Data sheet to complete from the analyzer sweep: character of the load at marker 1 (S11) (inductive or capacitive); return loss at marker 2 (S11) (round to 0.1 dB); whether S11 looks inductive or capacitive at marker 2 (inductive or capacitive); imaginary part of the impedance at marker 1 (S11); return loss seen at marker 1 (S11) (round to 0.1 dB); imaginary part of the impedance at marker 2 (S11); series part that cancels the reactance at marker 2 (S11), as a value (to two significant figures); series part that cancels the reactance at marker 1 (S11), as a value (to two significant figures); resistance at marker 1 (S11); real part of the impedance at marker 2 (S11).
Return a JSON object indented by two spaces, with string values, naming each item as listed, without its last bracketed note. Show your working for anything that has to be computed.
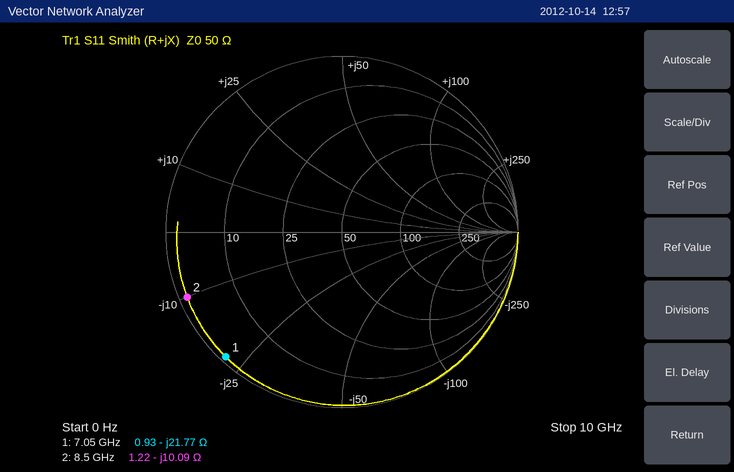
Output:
{
  "character of the load at marker 1 (S11)": "capacitive",
  "return loss at marker 2 (S11)": "0.4 dB",
  "whether S11 looks inductive or capacitive at marker 2": "capacitive",
  "imaginary part of the impedance at marker 1": "-21.77 Ω",
  "return loss seen at marker 1 (S11)": "0.3 dB",
  "imaginary part of the impedance at marker 2": "-10.09 Ω",
  "series part that cancels the reactance at marker 2 (S11), as a value": "L = 10.09 Ω/(2π × 8.5 GHz) ≈ 189 pH, so 190 pH to two significant figures",
  "series part that cancels the reactance at marker 1 (S11), as a value": "L = 21.77 Ω/(2π × 7.05 GHz) ≈ 491 pH, so 490 pH to two significant figures",
  "resistance at marker 1": "0.93 Ω",
  "real part of the impedance at marker 2": "1.22 Ω"
}
